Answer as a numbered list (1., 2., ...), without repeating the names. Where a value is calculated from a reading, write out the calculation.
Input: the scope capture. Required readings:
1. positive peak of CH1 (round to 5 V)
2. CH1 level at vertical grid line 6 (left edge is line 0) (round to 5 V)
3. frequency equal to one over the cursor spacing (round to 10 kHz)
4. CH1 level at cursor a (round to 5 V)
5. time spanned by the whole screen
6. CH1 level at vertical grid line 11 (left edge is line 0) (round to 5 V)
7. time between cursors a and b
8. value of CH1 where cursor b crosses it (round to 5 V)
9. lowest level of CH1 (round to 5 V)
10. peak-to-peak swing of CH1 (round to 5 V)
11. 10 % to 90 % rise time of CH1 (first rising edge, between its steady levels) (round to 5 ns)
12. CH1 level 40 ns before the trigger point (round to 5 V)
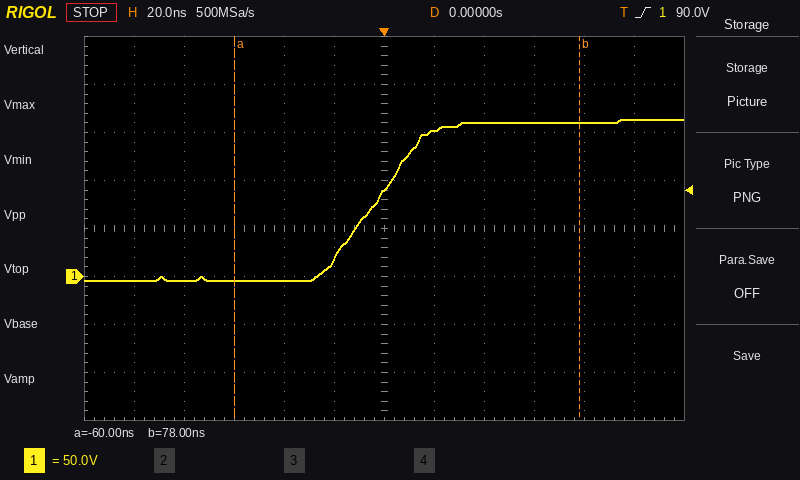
1. 165 V
2. 90 V
3. 1 / 138 ns ≈ 7.25 MHz
4. -5 V
5. 240 ns
6. 165 V
7. 78 ns − (-60 ns) = 138 ns
8. 160 V
9. -5 V
10. 165 V − (-5 V) = 170 V
11. 35 ns
12. -5 V
